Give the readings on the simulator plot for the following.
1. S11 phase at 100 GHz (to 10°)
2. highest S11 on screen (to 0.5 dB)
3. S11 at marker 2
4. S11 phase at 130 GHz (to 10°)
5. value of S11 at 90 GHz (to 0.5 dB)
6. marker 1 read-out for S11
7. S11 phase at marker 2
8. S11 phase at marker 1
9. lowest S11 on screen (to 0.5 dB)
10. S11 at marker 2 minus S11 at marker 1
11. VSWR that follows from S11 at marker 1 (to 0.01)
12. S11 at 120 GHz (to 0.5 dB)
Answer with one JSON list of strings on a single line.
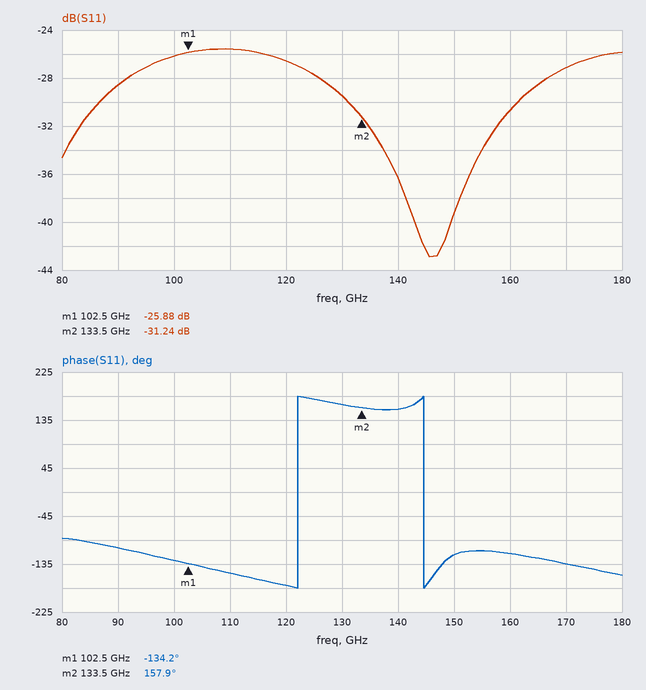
["-130°", "-25.5 dB", "-31.24 dB", "160°", "-28.5 dB", "-25.88 dB", "157.9°", "-134.2°", "-43.0 dB", "-5.36 dB", "1.11", "-26.5 dB"]
